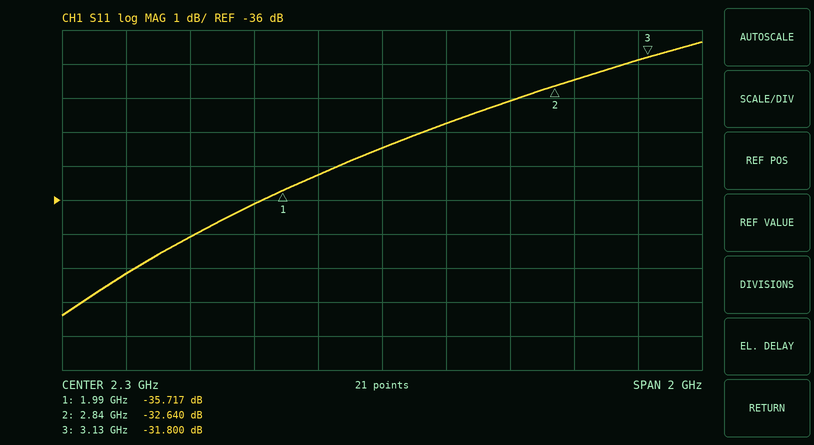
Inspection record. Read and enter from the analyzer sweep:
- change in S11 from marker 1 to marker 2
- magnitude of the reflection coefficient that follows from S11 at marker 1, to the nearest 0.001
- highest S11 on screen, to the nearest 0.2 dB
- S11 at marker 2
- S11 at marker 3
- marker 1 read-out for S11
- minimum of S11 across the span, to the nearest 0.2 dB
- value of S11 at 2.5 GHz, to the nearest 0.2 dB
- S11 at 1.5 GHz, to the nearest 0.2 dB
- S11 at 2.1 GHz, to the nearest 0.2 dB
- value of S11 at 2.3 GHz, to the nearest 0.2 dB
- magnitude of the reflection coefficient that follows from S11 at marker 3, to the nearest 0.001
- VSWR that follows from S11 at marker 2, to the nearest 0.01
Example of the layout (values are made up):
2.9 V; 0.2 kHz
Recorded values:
3.077 dB; 0.016; -31.4 dB; -32.640 dB; -31.800 dB; -35.717 dB; -39.4 dB; -33.8 dB; -38.2 dB; -35.2 dB; -34.4 dB; 0.026; 1.05
